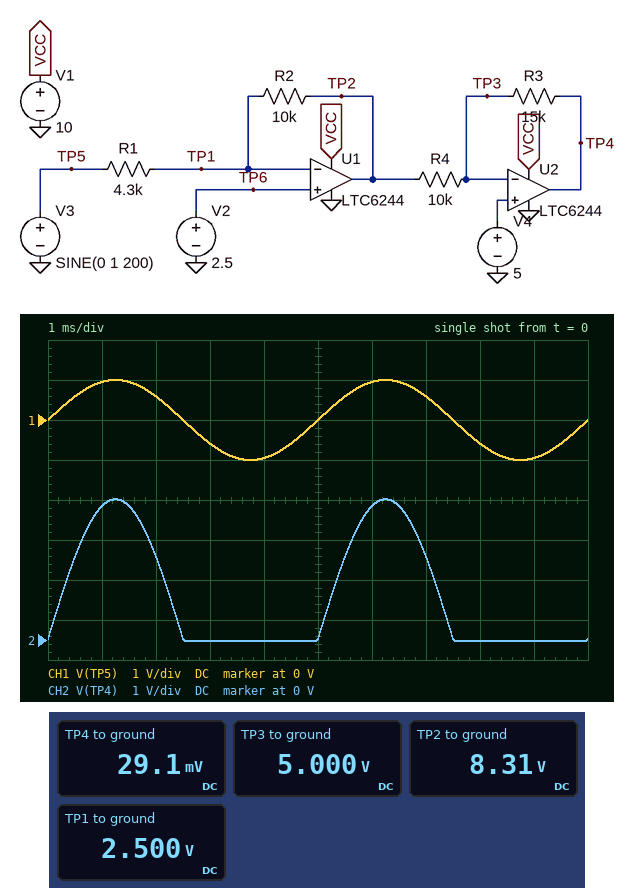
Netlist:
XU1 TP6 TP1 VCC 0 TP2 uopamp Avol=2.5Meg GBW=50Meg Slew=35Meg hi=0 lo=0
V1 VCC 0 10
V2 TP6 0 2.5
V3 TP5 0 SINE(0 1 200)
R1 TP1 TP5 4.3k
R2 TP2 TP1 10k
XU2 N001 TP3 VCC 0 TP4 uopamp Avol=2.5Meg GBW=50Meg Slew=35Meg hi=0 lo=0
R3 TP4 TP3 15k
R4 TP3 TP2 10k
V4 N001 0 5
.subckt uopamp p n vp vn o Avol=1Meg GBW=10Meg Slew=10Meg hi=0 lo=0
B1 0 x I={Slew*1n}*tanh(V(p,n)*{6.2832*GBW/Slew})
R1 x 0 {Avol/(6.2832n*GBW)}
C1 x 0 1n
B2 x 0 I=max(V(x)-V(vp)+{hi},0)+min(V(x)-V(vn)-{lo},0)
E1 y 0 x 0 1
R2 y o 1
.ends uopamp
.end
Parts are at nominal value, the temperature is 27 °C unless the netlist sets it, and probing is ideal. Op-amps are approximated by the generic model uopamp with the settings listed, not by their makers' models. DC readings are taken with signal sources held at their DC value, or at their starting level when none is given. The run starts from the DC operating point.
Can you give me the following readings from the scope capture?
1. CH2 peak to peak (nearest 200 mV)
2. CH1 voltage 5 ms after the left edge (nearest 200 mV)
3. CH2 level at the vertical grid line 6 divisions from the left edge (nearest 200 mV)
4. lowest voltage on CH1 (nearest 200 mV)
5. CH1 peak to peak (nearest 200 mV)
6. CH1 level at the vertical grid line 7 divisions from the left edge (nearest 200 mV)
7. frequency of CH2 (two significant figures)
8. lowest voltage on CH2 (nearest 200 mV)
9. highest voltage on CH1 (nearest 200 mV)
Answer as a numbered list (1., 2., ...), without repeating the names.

1. 3.6 V
2. 0 V
3. 3.4 V
4. -1.0 V
5. 2.0 V
6. 600 mV
7. 200 Hz
8. 0 V
9. 1.0 V
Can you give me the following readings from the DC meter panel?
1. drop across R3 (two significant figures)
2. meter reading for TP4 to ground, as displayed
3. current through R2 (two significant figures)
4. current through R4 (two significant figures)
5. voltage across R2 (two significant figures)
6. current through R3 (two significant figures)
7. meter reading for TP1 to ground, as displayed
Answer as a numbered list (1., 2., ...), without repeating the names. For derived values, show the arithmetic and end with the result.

1. 5 V - 29.1 mV = 5.0 V
2. 29.1 mV
3. (8.31 V - 2.5 V) / 10 kΩ = 580 µA
4. (8.31 V - 5 V) / 10 kΩ = 330 µA
5. 8.31 V - 2.5 V = 5.8 V
6. (5 V - 29.1 mV) / 15 kΩ = 330 µA
7. 2.500 V
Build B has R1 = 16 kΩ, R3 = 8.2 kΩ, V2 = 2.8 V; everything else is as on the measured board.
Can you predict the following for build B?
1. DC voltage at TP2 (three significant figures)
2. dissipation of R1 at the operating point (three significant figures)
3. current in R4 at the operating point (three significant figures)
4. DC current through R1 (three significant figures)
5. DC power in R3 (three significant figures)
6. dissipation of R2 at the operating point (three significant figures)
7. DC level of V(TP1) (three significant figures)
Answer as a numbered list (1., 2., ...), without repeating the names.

1. 4.55 V
2. 490 µW
3. 45.0 µA
4. 175 µA
5. 16.6 µW
6. 306 µW
7. 2.80 V
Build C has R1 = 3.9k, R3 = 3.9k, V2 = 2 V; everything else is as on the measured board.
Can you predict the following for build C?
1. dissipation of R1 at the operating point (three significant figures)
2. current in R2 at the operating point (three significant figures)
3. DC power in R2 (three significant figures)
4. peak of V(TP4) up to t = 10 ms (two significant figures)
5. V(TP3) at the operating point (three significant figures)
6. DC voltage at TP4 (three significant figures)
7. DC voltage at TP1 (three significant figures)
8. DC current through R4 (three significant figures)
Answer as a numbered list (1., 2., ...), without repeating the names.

1. 1.03 mW
2. 513 µA
3. 2.63 mW
4. 5.2 V
5. 5.00 V
6. 4.17 V
7. 2.00 V
8. 213 µA
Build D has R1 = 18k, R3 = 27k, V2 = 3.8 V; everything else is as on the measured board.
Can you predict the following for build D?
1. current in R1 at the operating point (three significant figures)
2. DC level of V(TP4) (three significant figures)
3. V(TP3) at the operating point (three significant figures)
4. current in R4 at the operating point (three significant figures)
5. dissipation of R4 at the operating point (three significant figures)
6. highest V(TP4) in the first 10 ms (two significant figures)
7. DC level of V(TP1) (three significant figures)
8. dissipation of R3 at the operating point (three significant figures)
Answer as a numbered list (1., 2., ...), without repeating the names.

1. 211 µA
2. 2.54 V
3. 5.00 V
4. 91.1 µA
5. 83.0 µW
6. 4.0 V
7. 3.80 V
8. 224 µW
